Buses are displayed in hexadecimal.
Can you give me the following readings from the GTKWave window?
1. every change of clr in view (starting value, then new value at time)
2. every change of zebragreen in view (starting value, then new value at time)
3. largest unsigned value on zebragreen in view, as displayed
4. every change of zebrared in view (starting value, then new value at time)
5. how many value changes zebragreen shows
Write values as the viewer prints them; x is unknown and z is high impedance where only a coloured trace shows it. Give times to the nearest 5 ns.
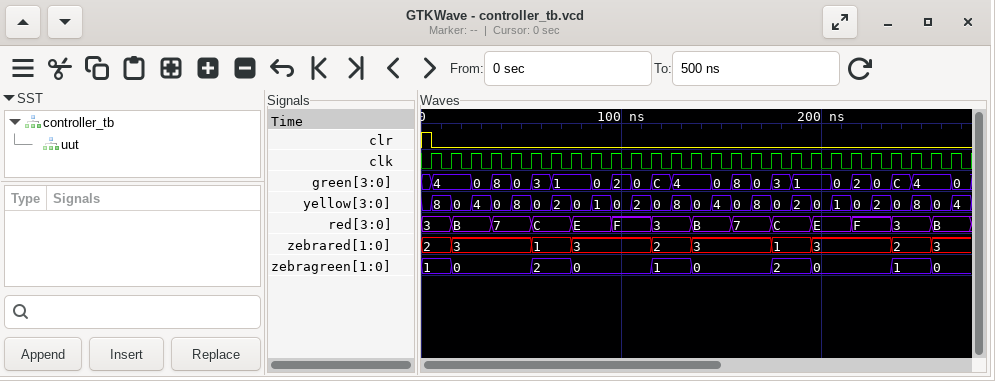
1, 0 at 5 ns
1, 0 at 15 ns, 2 at 55 ns, 0 at 75 ns, 1 at 115 ns, 0 at 135 ns, 2 at 175 ns, 0 at 195 ns, 1 at 235 ns, 0 at 255 ns
2
2, 3 at 15 ns, 1 at 55 ns, 3 at 75 ns, 2 at 115 ns, 3 at 135 ns, 1 at 175 ns, 3 at 195 ns, 2 at 235 ns, 3 at 255 ns
9
